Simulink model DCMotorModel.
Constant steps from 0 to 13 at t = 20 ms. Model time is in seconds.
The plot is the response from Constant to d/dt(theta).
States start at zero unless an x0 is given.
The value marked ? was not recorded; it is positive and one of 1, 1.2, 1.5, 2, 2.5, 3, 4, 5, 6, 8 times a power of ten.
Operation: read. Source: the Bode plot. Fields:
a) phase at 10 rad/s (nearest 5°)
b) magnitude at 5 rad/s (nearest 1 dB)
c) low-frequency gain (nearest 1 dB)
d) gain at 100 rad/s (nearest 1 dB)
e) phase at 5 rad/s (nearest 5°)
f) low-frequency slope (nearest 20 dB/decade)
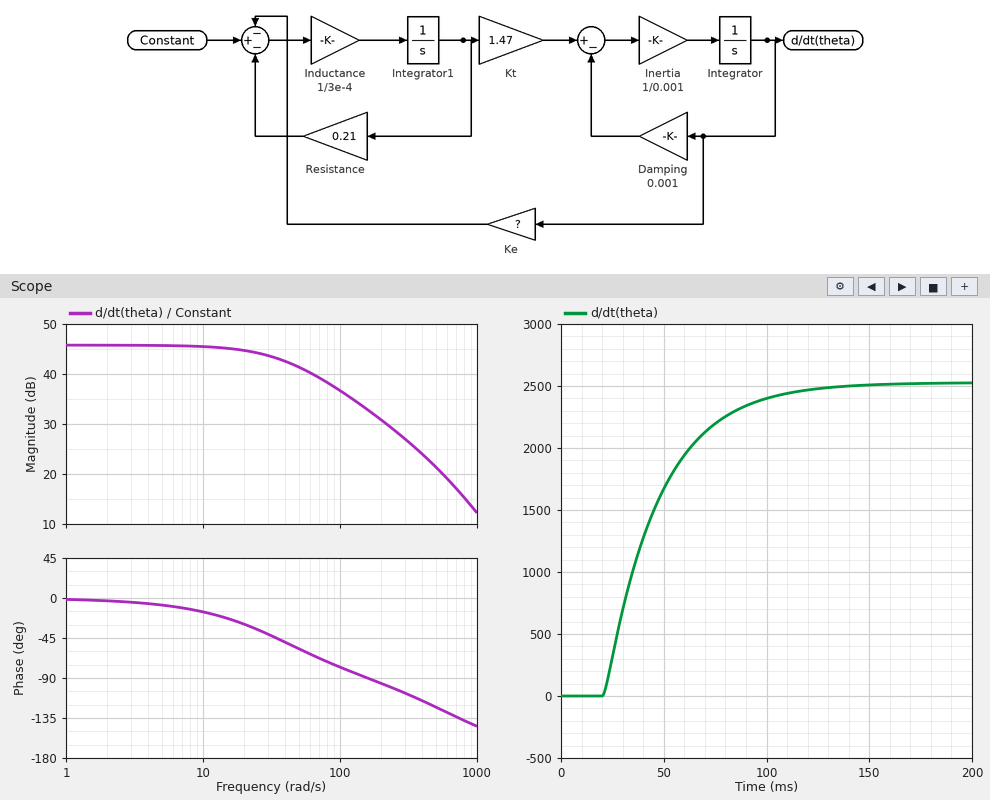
-15°
46 dB
46 dB
37 dB
-10°
0 dB/decade
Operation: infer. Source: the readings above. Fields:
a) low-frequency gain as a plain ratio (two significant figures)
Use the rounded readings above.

200
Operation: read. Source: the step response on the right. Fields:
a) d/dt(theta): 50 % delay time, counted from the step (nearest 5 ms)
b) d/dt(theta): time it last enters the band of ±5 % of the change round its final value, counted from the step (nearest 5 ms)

20 ms
80 ms
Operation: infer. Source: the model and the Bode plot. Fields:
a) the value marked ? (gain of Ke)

0.005
